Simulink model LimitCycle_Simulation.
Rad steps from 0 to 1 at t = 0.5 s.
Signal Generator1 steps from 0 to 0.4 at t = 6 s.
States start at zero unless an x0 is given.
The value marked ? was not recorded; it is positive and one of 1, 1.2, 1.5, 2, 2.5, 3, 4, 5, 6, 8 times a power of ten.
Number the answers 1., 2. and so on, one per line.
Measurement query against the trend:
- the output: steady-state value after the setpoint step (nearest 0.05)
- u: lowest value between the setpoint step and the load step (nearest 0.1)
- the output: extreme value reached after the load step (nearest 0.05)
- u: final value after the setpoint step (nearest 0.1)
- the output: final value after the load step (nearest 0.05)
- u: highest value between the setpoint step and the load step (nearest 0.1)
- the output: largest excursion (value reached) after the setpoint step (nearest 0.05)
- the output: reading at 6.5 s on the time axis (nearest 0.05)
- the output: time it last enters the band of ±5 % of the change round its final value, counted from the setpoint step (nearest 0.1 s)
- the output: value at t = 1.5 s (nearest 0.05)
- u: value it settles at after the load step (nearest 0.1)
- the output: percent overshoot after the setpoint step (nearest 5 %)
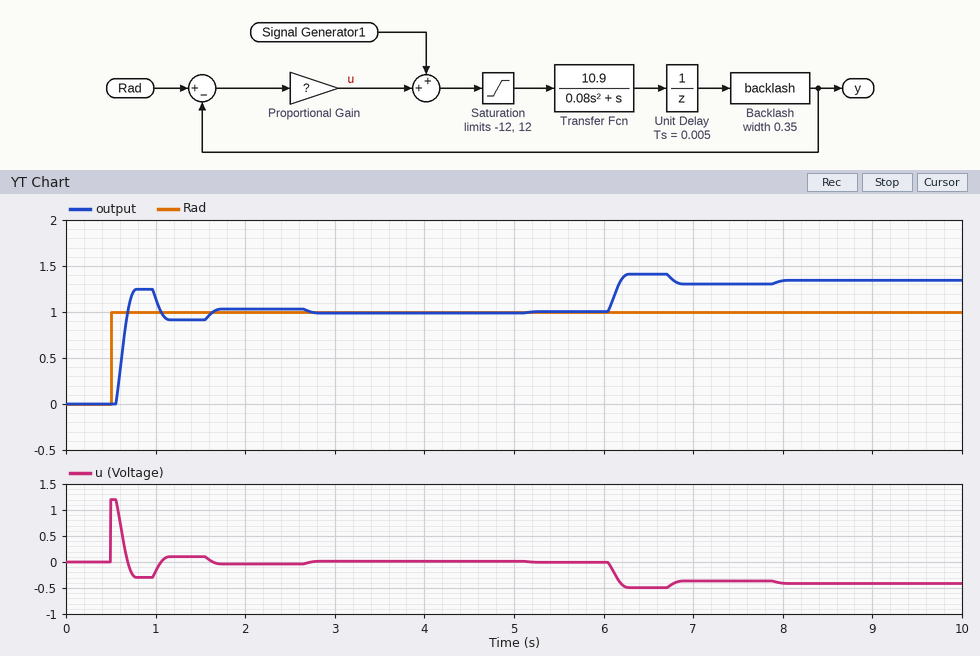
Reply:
1. 1.00
2. -0.3
3. 1.40
4. 0.0
5. 1.35
6. 1.2
7. 1.25
8. 1.40
9. 1.1 s
10. 0.90
11. -0.4
12. 25 %
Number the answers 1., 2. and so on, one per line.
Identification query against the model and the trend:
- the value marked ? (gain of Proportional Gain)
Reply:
1. 1.2
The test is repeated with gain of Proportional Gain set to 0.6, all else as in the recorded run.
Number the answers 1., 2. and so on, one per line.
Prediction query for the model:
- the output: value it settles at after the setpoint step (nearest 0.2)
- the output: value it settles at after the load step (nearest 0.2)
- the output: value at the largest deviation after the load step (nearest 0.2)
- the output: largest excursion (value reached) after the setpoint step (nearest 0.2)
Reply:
1. 1.0
2. 1.6
3. 1.8
4. 1.0
